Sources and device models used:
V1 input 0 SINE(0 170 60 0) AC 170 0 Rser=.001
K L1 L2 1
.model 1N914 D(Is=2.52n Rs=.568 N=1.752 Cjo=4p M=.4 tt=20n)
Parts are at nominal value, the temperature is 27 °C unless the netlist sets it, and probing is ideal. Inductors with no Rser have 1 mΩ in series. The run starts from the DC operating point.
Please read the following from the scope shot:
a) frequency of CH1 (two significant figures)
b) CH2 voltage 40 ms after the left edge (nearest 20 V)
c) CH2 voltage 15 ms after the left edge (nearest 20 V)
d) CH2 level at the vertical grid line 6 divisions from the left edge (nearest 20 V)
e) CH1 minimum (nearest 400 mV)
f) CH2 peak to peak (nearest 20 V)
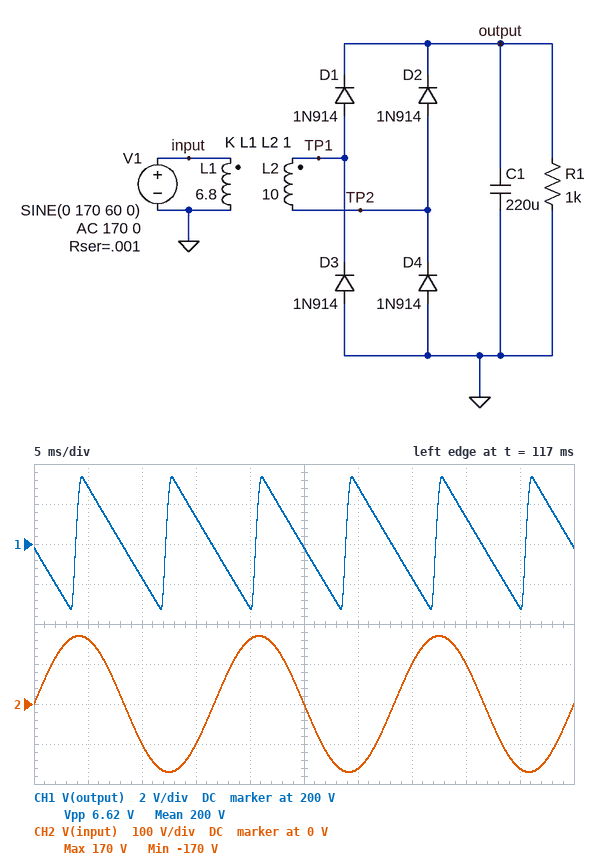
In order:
120 Hz
100 V
-100 V
-160 V
196.8 V
340 V
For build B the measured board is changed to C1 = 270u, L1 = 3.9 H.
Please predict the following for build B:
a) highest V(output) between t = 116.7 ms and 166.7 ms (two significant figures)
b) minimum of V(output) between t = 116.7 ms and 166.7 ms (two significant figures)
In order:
270 V
260 V
